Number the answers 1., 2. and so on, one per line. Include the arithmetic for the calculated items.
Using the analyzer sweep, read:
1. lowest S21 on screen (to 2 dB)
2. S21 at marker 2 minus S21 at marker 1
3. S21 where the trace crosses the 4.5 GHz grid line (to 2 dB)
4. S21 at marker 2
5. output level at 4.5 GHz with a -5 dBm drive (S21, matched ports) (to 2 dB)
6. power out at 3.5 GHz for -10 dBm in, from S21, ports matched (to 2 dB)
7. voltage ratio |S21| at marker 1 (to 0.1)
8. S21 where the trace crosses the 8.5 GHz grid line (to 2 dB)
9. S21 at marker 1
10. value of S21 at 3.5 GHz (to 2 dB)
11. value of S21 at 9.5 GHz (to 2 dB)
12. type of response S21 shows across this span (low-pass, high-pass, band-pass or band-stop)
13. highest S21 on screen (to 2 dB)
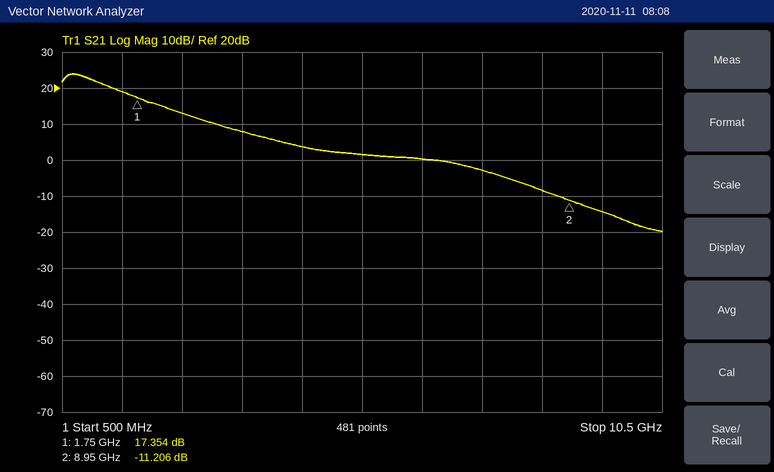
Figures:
1. -20 dB
2. -11.206 − (17.354) = -28.560 dB
3. 4 dB
4. -11.206 dB
5. -5 dBm + (4 dB) = -2 dBm
6. -10 dBm + (8 dB) = -2 dBm
7. 10^(17.354/20) ≈ 7.4
8. -8 dB
9. 17.354 dB
10. 8 dB
11. -14 dB
12. low-pass
13. 24 dB
